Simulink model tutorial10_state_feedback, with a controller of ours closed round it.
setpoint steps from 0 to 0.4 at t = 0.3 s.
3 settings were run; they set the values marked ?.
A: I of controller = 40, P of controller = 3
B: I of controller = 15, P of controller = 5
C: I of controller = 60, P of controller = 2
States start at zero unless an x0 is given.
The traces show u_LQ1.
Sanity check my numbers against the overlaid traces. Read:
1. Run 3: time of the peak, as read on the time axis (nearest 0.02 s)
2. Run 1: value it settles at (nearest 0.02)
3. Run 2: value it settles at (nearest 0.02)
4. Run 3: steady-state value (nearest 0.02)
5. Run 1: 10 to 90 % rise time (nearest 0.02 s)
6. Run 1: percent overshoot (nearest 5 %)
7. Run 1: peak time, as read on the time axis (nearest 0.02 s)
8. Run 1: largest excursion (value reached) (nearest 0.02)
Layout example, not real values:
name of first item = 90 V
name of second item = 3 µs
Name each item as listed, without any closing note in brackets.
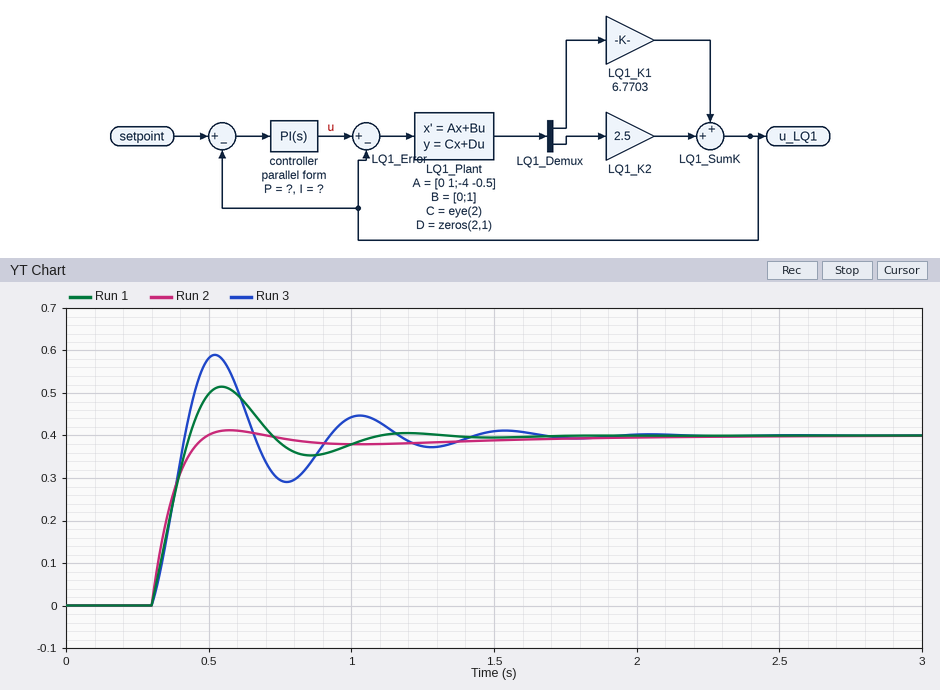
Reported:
Run 3: time of the peak, as read on the time axis = 0.52 s
Run 1: value it settles at = 0.40
Run 2: value it settles at = 0.40
Run 3: steady-state value = 0.40
Run 1: 10 to 90 % rise time = 0.10 s
Run 1: percent overshoot = 30 %
Run 1: peak time, as read on the time axis = 0.54 s
Run 1: largest excursion (value reached) = 0.52
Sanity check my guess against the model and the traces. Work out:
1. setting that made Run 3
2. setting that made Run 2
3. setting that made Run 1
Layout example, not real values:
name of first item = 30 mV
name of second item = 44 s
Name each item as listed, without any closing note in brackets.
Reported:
setting that made Run 3 = C
setting that made Run 2 = B
setting that made Run 1 = A
